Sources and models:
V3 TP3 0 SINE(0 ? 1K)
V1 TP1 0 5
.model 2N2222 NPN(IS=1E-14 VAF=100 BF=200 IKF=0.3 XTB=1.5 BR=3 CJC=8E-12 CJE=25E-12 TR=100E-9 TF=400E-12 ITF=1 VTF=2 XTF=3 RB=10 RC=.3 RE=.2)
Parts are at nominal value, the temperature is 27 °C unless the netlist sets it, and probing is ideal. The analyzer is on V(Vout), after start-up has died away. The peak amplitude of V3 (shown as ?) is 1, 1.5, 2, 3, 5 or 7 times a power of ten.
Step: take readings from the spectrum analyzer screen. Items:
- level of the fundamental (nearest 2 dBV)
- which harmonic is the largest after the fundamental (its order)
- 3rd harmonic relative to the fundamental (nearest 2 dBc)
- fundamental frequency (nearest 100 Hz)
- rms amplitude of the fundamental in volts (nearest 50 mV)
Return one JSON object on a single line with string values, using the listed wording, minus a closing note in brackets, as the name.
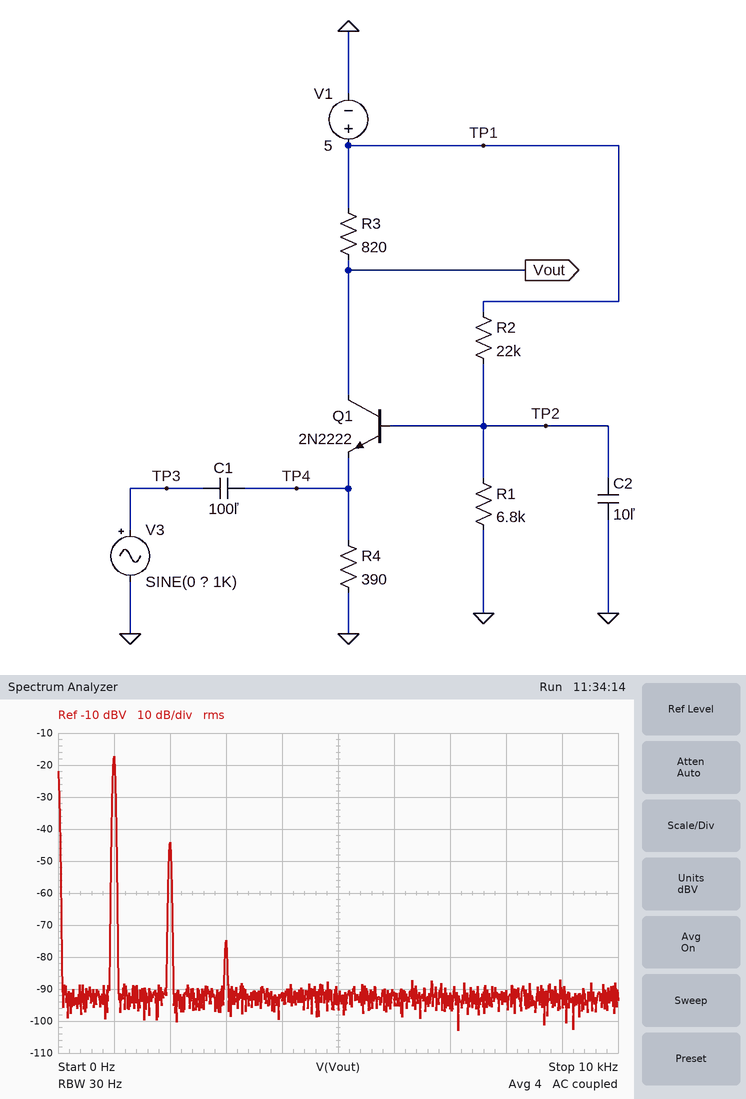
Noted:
{"level of the fundamental": "-18 dBV", "which harmonic is the largest after the fundamental": "2", "3rd harmonic relative to the fundamental": "-58 dBc", "fundamental frequency": "1.0 kHz", "rms amplitude of the fundamental in volts": "150 mV"}
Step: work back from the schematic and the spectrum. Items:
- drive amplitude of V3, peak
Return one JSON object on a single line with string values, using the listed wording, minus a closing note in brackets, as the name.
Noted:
{"drive amplitude of V3, peak": "5 mV"}
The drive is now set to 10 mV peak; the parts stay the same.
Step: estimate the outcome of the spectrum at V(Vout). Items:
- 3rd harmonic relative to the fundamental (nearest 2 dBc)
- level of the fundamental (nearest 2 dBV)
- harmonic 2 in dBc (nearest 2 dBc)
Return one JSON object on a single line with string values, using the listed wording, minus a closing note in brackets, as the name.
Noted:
{"3rd harmonic relative to the fundamental": "-46 dBc", "level of the fundamental": "-12 dBV", "harmonic 2 in dBc": "-20 dBc"}
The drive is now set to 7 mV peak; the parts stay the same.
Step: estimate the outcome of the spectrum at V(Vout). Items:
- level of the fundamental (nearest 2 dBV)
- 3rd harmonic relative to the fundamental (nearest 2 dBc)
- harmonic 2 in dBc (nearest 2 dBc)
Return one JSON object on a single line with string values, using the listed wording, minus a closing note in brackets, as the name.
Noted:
{"level of the fundamental": "-14 dBV", "3rd harmonic relative to the fundamental": "-52 dBc", "harmonic 2 in dBc": "-24 dBc"}
